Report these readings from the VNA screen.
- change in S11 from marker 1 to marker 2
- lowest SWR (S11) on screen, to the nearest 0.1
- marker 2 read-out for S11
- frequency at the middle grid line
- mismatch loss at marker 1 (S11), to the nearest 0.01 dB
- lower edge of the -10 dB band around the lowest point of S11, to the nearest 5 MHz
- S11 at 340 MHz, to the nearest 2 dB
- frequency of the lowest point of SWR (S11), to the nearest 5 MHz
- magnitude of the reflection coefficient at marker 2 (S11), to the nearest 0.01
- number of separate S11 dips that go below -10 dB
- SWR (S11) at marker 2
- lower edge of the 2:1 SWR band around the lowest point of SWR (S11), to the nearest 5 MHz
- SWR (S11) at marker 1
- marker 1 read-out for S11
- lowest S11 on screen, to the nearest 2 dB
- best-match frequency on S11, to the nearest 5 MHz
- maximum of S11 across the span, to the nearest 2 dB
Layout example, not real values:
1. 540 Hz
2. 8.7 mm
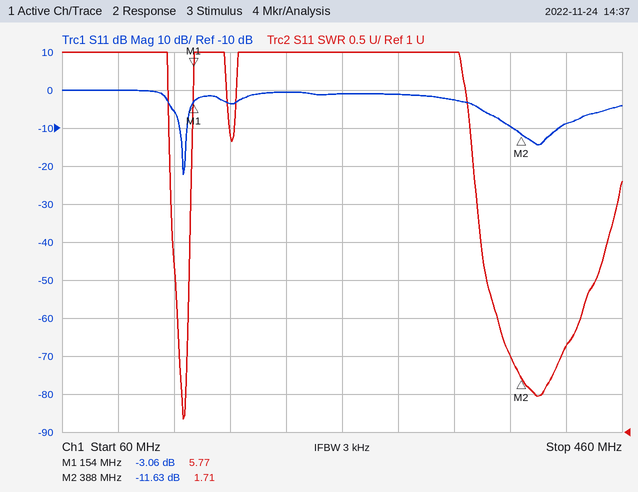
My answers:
1. -8.57 dB
2. 1.2
3. -11.63 dB
4. 260 MHz
5. 2.96 dB
6. 145 MHz
7. -2 dB
8. 145 MHz
9. 0.26
10. 2
11. 1.71
12. 145 MHz
13. 5.77
14. -3.06 dB
15. -22 dB
16. 145 MHz
17. 0 dB
